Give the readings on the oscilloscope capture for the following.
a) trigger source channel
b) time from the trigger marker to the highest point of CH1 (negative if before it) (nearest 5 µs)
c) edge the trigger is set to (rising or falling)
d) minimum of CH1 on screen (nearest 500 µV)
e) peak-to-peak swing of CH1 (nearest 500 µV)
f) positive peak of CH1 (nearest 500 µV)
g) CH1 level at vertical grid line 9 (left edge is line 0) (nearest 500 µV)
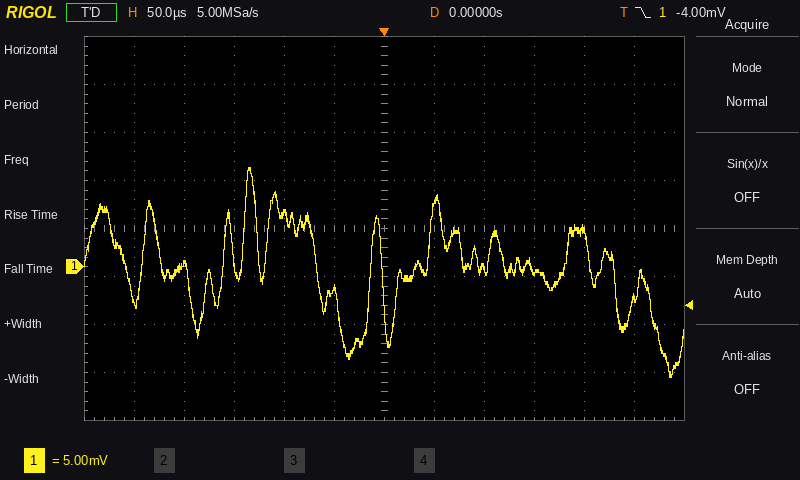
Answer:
CH1
-135 µs
falling
-11.5 mV
22.0 mV
10.5 mV
-500 µV
